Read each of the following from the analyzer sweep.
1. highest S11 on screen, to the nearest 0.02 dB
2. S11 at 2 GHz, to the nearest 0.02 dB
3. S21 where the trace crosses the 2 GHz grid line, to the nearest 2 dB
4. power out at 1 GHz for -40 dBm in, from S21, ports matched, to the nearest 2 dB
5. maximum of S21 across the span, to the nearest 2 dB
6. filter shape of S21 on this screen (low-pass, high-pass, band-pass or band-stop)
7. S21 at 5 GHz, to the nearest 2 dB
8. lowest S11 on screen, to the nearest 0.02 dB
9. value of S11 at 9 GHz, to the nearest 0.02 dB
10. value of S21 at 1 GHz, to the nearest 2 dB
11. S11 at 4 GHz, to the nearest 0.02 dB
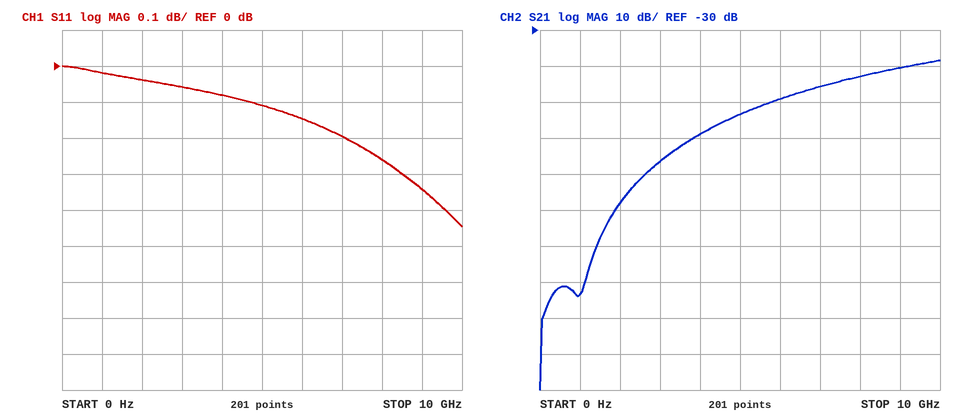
0.00 dB
-0.04 dB
-78 dB
-144 dBm
-38 dB
high-pass
-54 dB
-0.44 dB
-0.34 dB
-104 dB
-0.08 dB
